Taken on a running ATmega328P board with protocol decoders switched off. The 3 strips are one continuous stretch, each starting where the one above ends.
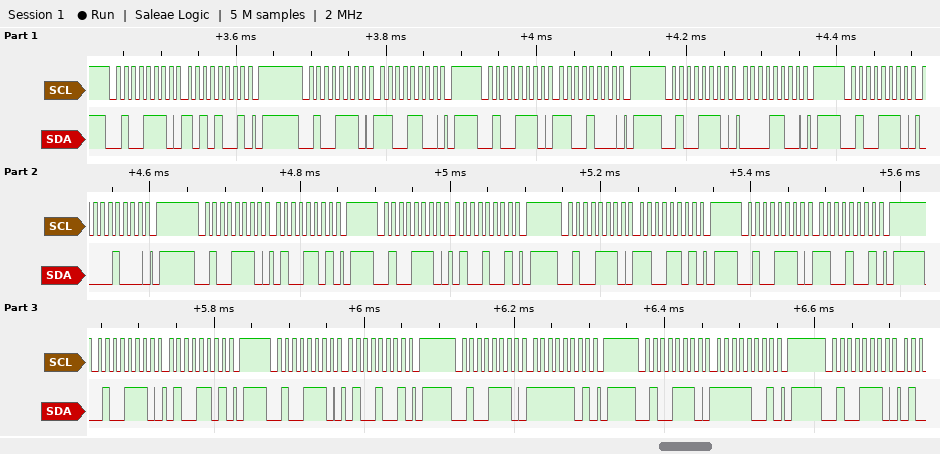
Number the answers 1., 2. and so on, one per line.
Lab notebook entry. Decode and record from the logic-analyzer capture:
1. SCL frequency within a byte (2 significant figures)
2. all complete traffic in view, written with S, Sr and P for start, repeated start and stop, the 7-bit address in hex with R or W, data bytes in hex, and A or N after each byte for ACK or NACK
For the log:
1. 100 kHz
2. S 27W A A9 A P S 27W A CC A P S 27W A C8 A P S 27W A 0C A P S 27W A 08 A P S 27W A 4D A P S 27W A 49 A P S 27W A CD A P S 27W A C9 A P S 27W A 4D A P S 27W A 49 A P S 27W A FD A P S 27W A F9 A P S 27W A
